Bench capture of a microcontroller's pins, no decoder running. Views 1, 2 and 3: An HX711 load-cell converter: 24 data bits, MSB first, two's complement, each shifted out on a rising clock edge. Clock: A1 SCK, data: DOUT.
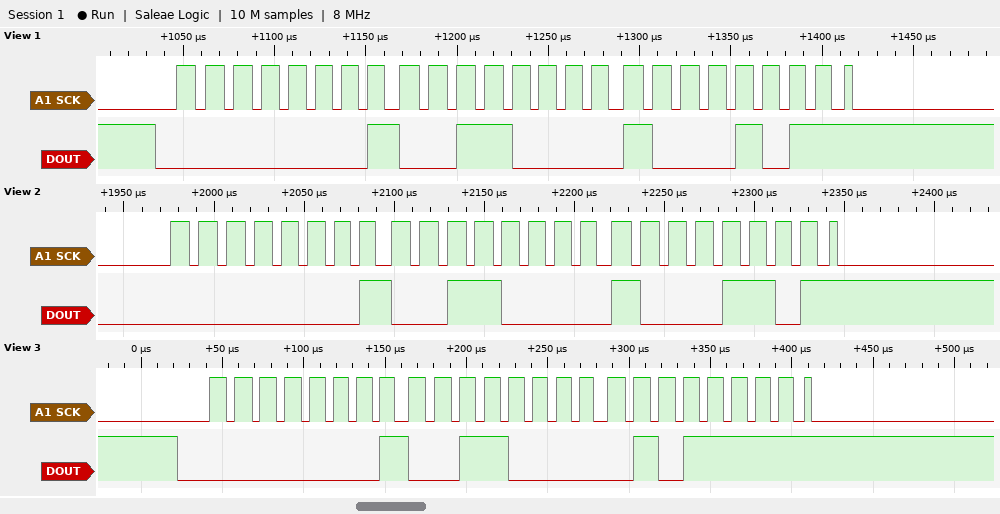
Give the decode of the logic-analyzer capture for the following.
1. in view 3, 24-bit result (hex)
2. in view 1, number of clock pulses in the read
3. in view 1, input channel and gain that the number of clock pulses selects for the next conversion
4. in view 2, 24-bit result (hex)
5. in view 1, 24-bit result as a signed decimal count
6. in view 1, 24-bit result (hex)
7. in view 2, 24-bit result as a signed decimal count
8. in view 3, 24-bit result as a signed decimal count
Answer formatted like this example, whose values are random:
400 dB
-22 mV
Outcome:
0x01305F
25
channel A, gain 128
0x01308D
77963
0x01308B
77965
77919
